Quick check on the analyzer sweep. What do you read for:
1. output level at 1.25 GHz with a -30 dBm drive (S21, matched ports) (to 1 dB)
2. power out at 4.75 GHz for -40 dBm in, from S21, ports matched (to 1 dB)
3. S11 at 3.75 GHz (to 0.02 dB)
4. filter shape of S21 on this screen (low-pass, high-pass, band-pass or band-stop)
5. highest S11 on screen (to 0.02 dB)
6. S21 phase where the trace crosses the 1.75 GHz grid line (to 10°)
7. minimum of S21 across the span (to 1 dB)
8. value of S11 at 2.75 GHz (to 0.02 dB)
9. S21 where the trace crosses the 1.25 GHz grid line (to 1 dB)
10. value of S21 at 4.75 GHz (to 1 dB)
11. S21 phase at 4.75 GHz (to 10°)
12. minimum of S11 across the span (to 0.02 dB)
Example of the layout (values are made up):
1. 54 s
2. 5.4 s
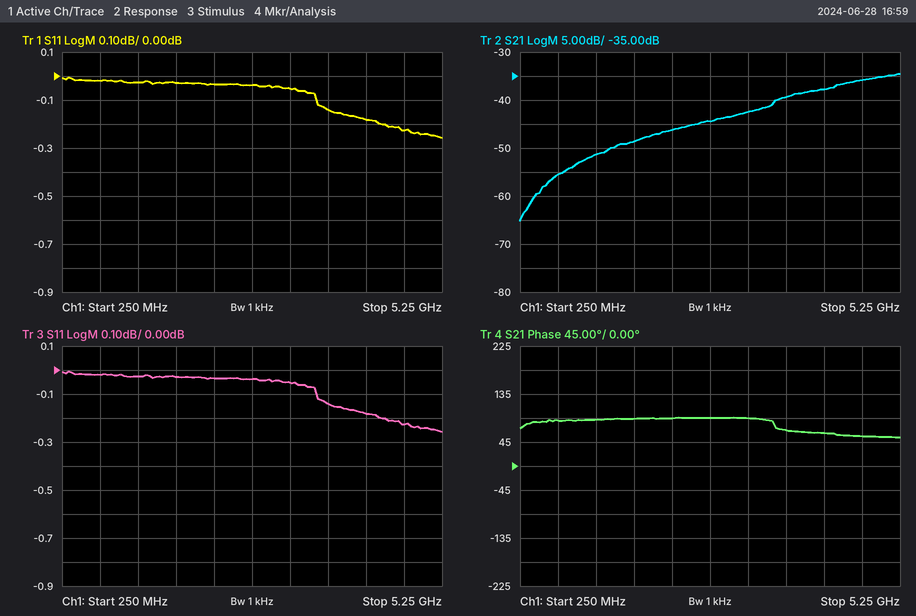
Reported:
1. -81 dBm
2. -76 dBm
3. -0.14 dB
4. high-pass
5. 0.00 dB
6. 90°
7. -65 dB
8. -0.04 dB
9. -51 dB
10. -36 dB
11. 60°
12. -0.26 dB
